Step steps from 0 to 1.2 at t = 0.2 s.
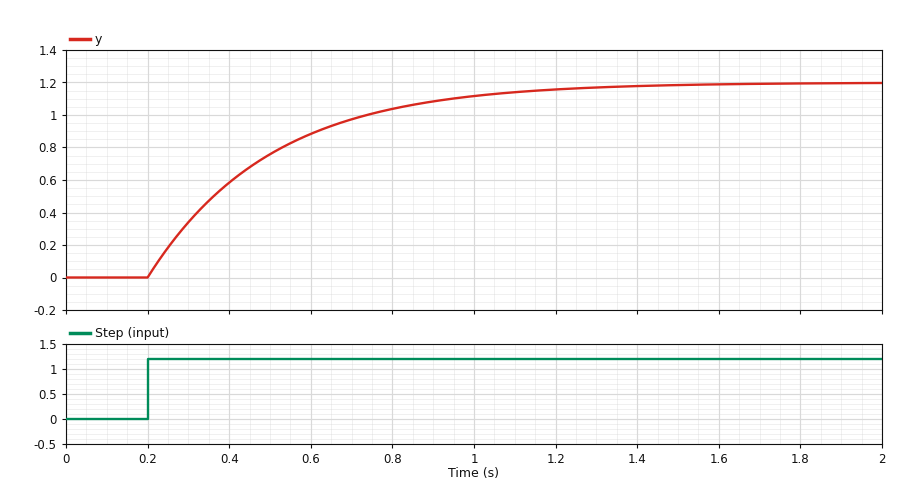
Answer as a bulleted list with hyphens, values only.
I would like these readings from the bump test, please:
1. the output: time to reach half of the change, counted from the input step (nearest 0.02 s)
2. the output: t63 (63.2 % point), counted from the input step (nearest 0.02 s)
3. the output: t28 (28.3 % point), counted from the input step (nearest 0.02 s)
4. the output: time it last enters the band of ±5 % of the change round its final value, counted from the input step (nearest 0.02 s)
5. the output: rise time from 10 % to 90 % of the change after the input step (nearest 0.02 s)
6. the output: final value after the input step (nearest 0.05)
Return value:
- 0.20 s
- 0.30 s
- 0.10 s
- 0.90 s
- 0.66 s
- 1.20
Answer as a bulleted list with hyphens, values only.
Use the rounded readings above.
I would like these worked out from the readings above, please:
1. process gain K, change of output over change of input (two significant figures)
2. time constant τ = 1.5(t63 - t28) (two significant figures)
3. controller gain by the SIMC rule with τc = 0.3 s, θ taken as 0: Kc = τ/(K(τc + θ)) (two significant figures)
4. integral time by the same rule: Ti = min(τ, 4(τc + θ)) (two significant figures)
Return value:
- 1.0
- 0.30 s
- 1.0
- 0.30 s
